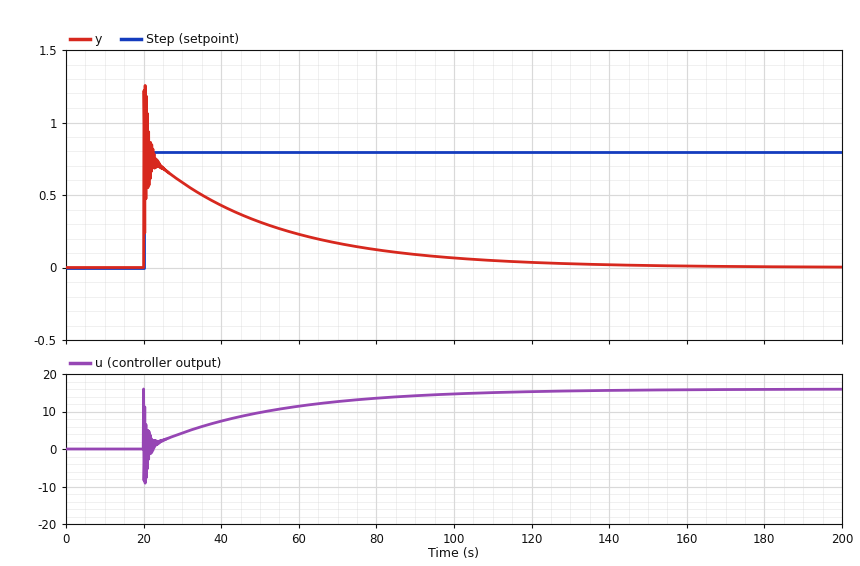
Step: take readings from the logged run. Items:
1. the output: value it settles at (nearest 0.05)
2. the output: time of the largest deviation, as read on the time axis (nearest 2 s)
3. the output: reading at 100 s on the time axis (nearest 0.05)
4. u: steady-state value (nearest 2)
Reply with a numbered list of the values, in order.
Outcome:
1. 0.00
2. 20 s
3. 0.05
4. 16
